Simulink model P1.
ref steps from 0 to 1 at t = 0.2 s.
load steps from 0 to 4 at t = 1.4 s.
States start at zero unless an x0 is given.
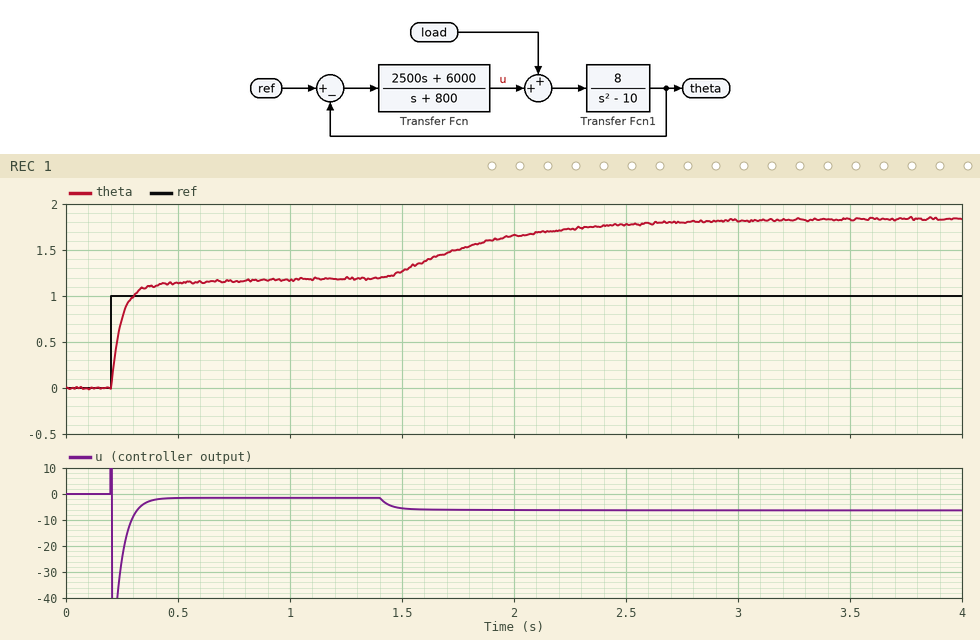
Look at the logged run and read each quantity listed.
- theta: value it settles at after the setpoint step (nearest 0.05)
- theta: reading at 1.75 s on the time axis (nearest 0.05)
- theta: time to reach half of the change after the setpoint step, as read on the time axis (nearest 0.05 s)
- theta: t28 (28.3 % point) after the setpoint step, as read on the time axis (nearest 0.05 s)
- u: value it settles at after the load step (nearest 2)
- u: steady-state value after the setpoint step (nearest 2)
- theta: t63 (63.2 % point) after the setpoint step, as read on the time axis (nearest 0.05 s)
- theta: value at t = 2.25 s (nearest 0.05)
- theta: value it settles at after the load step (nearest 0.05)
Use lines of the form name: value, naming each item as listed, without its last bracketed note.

theta: value it settles at after the setpoint step: 1.20
theta: reading at 1.75 s on the time axis: 1.50
theta: time to reach half of the change after the setpoint step, as read on the time axis: 0.25 s
theta: t28 (28.3 % point) after the setpoint step, as read on the time axis: 0.20 s
u: value it settles at after the load step: -6
u: steady-state value after the setpoint step: -2
theta: t63 (63.2 % point) after the setpoint step, as read on the time axis: 0.25 s
theta: value at t = 2.25 s: 1.75
theta: value it settles at after the load step: 1.85
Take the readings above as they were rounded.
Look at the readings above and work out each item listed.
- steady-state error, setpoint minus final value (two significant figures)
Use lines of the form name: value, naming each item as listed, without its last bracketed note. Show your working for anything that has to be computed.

steady-state error, setpoint minus final value: 1 - 1.2 = -0.20
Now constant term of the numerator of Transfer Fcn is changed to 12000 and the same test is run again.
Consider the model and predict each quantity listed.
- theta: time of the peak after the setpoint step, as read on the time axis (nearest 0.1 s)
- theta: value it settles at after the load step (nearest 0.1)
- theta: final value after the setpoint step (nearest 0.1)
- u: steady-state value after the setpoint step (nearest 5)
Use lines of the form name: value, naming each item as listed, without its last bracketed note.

theta: time of the peak after the setpoint step, as read on the time axis: 0.4 s
theta: value it settles at after the load step: 1.4
theta: final value after the setpoint step: 1.1
u: steady-state value after the setpoint step: 0
